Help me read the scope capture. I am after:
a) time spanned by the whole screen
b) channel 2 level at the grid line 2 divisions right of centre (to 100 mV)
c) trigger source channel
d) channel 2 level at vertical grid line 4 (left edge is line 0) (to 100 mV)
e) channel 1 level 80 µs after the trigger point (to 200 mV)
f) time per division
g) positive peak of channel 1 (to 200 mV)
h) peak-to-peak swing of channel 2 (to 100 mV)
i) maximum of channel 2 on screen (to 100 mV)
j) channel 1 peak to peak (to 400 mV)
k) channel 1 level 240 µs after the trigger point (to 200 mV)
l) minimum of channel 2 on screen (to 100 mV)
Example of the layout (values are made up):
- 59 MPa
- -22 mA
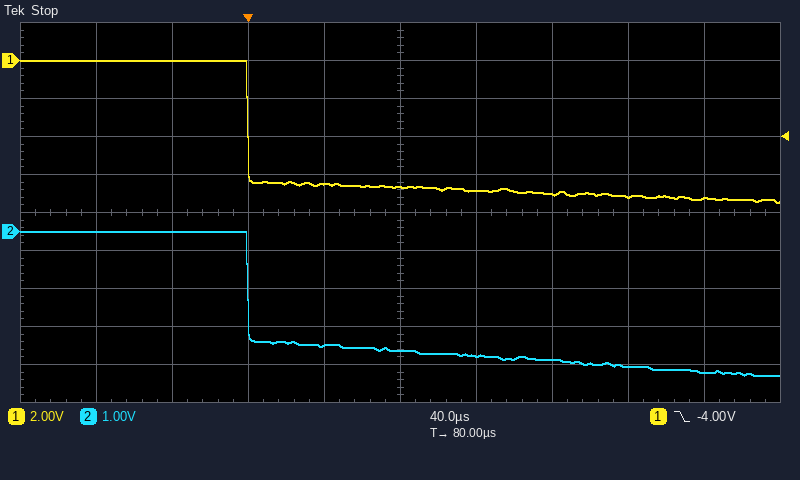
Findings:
- 400 µs
- -3.4 V
- channel 1
- -3.0 V
- -6.6 V
- 40 µs
- 0.0 V
- 3.8 V
- 0.0 V
- 7.6 V
- -7.2 V
- -3.8 V
